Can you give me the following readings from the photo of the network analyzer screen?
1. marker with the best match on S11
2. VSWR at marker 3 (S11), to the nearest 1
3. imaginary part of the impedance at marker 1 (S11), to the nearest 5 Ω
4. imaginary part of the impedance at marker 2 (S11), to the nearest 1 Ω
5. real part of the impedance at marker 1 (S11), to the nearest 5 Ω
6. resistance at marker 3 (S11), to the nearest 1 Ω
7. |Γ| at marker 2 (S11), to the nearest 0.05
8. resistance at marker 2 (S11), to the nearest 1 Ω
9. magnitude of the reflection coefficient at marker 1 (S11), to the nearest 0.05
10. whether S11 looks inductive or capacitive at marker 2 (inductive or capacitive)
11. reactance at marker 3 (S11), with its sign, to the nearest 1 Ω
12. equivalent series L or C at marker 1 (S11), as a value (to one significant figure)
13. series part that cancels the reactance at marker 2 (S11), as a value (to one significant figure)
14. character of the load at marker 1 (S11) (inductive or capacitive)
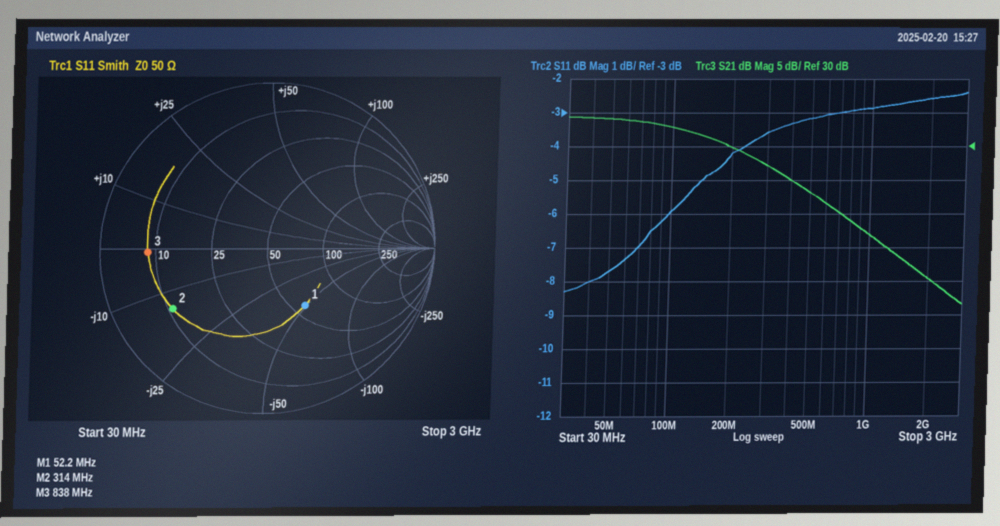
marker 1
6
-50 Ω
-14 Ω
60 Ω
8 Ω
0.65
11 Ω
0.40
capacitive
-1 Ω
60 pF
7 nH
capacitive
